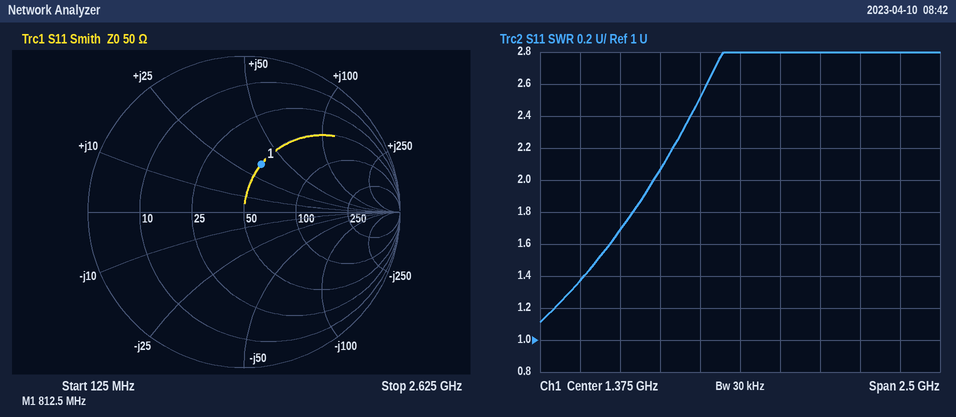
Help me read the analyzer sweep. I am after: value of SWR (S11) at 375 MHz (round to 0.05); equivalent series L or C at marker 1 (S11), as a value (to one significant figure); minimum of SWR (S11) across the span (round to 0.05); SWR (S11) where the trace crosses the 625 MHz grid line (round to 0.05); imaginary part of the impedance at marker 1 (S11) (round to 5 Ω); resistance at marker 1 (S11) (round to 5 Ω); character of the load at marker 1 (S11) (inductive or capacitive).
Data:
1.35
7 nH
1.10
1.70
+35 Ω
50 Ω
inductive
